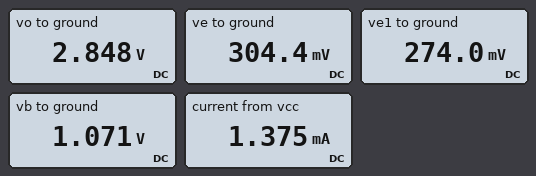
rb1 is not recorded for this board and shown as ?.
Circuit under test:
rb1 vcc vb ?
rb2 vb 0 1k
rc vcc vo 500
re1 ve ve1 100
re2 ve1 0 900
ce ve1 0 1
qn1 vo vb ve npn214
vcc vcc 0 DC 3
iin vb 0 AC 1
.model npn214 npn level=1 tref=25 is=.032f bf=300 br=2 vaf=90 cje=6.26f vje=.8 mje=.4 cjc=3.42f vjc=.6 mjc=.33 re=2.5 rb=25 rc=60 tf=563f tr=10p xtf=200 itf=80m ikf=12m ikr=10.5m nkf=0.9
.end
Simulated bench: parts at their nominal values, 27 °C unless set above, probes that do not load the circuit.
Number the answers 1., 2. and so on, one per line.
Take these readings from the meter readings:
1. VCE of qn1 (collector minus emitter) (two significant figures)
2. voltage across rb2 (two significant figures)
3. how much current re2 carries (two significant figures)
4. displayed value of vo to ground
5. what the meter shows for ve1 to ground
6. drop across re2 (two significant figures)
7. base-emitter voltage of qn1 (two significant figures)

1. 2.5 V
2. 1.1 V
3. 300 µA
4. 2.848 V
5. 274.0 mV
6. 270 mV
7. 770 mV
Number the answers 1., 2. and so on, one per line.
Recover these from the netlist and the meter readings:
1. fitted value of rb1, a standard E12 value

1. 1.8 kΩ
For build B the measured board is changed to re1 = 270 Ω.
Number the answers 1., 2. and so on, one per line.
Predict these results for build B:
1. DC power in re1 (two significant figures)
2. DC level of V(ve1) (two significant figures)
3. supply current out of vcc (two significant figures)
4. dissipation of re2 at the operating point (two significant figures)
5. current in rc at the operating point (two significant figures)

1. 19 µW
2. 240 mV
3. 1.3 mA
4. 63 µW
5. 260 µA
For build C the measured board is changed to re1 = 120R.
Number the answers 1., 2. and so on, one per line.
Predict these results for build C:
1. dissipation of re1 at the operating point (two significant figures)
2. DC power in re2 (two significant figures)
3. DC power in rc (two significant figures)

1. 11 µW
2. 80 µW
3. 44 µW
